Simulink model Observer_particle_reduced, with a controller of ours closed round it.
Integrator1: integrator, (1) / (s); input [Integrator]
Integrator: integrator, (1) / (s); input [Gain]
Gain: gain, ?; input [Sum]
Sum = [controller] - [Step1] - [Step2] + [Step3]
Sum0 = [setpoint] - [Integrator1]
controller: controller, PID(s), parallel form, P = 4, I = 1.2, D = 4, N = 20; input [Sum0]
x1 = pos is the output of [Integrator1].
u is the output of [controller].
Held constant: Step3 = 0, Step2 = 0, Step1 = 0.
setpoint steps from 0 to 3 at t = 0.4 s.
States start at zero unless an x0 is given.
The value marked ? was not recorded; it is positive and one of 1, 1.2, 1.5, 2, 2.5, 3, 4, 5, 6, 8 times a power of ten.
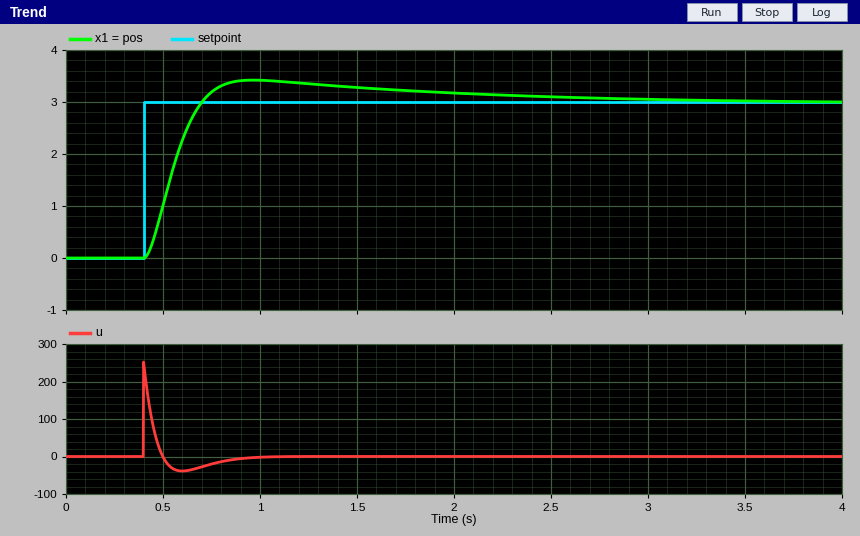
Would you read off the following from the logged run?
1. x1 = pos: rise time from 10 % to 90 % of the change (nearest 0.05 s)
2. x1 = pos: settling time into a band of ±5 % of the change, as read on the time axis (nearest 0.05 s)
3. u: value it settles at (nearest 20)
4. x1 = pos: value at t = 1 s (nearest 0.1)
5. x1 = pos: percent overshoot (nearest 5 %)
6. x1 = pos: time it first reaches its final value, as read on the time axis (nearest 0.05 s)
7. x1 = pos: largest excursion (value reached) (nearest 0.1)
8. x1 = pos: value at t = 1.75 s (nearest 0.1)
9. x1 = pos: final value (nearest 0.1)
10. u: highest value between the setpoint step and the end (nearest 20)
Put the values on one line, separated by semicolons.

0.20 s; 2.15 s; 0; 3.4; 15 %; 0.70 s; 3.4; 3.2; 3.0; 260
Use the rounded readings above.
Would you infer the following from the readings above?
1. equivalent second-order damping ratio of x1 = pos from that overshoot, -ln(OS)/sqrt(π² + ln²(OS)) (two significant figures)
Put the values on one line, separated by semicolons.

0.52
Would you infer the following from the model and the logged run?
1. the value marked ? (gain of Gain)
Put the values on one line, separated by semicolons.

1.5
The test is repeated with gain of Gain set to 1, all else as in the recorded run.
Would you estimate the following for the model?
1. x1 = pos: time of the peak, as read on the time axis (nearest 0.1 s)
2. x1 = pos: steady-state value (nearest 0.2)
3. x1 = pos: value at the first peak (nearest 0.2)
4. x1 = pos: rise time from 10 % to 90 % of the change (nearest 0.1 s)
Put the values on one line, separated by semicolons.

1.3 s; 3.0; 3.6; 0.3 s
